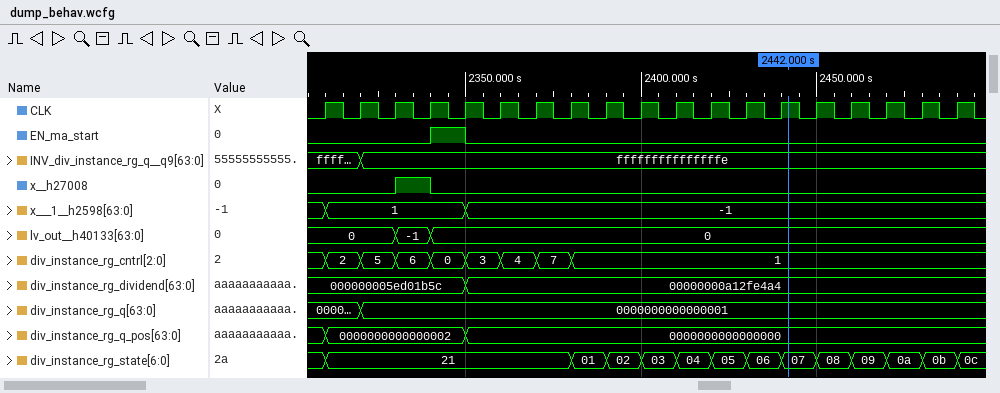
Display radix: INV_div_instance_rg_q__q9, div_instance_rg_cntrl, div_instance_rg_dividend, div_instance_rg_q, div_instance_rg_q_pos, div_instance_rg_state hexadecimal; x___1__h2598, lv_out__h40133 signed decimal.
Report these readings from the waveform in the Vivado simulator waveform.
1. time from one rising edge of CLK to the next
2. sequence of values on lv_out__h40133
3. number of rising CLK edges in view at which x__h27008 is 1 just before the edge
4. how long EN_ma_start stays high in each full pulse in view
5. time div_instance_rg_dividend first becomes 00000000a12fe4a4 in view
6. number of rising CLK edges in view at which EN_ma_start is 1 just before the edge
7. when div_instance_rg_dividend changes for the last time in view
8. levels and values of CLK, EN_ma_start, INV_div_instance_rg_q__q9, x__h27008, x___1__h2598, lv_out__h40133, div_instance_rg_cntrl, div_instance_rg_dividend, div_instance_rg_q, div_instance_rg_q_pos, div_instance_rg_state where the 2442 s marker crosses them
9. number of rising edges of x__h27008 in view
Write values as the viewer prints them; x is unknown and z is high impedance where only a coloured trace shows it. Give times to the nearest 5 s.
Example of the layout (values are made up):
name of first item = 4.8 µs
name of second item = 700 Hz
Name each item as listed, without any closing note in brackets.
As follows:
time from one rising edge of CLK to the next = 10 s
sequence of values on lv_out__h40133 = 0, -1, 0
number of rising CLK edges in view at which x__h27008 is 1 just before the edge = 1
how long EN_ma_start stays high in each full pulse in view = 10 s
time div_instance_rg_dividend first becomes 00000000a12fe4a4 in view = 2350 s
number of rising CLK edges in view at which EN_ma_start is 1 just before the edge = 1
when div_instance_rg_dividend changes for the last time in view = 2350 s
levels and values of CLK, EN_ma_start, INV_div_instance_rg_q__q9, x__h27008, x___1__h2598, lv_out__h40133, div_instance_rg_cntrl, div_instance_rg_dividend, div_instance_rg_q, div_instance_rg_q_pos, div_instance_rg_state where the 2442 s marker crosses them = CLK=1, EN_ma_start=0, INV_div_instance_rg_q__q9=fffffffffffffffe, x__h27008=0, x___1__h2598=-1, lv_out__h40133=0, div_instance_rg_cntrl=1, div_instance_rg_dividend=00000000a12fe4a4, div_instance_rg_q=0000000000000001, div_instance_rg_q_pos=0000000000000000, div_instance_rg_state=07
number of rising edges of x__h27008 in view = 1
